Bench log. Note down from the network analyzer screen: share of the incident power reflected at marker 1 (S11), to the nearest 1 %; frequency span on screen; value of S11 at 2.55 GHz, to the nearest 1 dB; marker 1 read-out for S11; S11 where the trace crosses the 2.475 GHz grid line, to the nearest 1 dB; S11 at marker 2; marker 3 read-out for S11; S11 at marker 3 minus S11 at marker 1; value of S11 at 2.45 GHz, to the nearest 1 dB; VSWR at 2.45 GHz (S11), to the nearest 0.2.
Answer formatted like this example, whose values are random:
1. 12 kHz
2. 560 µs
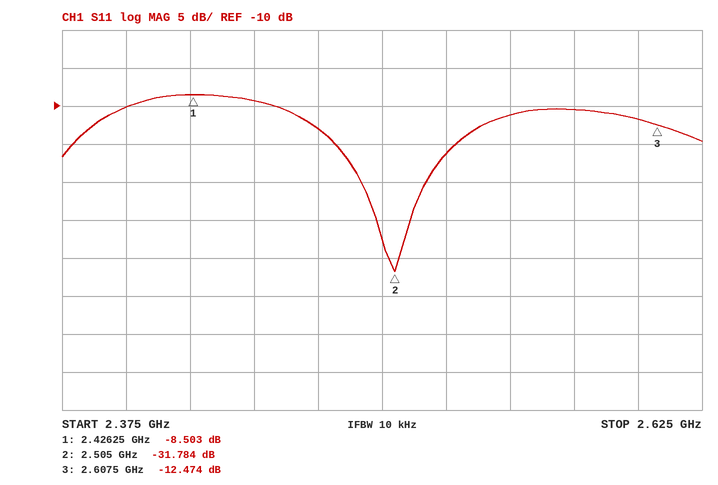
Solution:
1. 14 %
2. 250 MHz
3. -11 dB
4. -8.503 dB
5. -13 dB
6. -31.784 dB
7. -12.474 dB
8. -3.971 dB
9. -9 dB
10. 2.0
